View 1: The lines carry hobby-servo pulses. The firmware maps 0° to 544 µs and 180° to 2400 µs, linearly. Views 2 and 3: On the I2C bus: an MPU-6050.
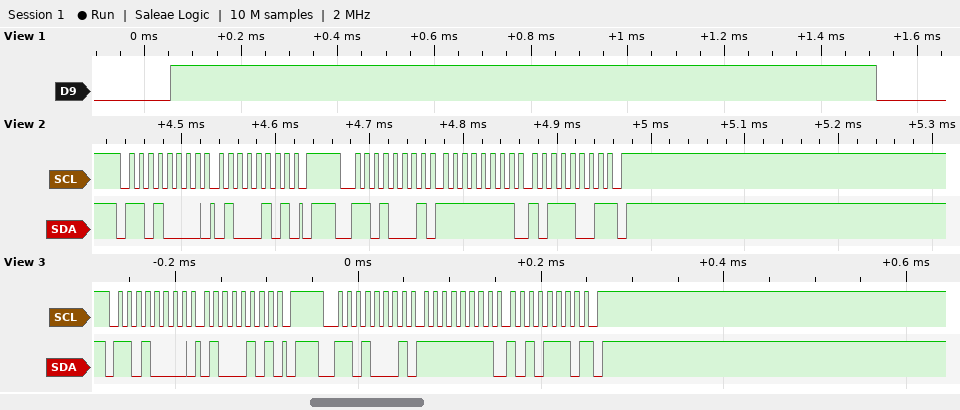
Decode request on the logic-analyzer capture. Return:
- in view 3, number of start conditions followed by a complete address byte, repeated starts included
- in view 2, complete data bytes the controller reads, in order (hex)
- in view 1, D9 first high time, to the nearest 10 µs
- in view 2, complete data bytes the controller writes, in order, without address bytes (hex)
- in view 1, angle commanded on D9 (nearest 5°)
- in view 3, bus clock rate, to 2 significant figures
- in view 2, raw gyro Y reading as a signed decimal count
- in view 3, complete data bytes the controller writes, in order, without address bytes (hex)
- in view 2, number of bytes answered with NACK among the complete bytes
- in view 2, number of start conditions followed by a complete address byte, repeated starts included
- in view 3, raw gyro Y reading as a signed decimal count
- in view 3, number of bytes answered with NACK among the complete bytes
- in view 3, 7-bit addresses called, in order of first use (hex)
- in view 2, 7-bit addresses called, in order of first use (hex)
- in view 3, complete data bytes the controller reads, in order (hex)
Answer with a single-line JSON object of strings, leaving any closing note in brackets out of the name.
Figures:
{"in view 3, number of start conditions followed by a complete address byte, repeated starts included": "2", "in view 2, complete data bytes the controller reads, in order": "FF B9", "in view 1, D9 first high time, to the nearest 10 µs": "1460 µs", "in view 2, complete data bytes the controller writes, in order, without address bytes": "45", "in view 1, angle commanded on D9": "90°", "in view 3, bus clock rate, to 2 significant figures": "100 kHz", "in view 2, raw gyro Y reading as a signed decimal count": "-71", "in view 3, complete data bytes the controller writes, in order, without address bytes": "45", "in view 2, number of bytes answered with NACK among the complete bytes": "1", "in view 2, number of start conditions followed by a complete address byte, repeated starts included": "2", "in view 3, raw gyro Y reading as a signed decimal count": "-82", "in view 3, number of bytes answered with NACK among the complete bytes": "1", "in view 3, 7-bit addresses called, in order of first use": "0x68", "in view 2, 7-bit addresses called, in order of first use": "0x68", "in view 3, complete data bytes the controller reads, in order": "FF AE"}
